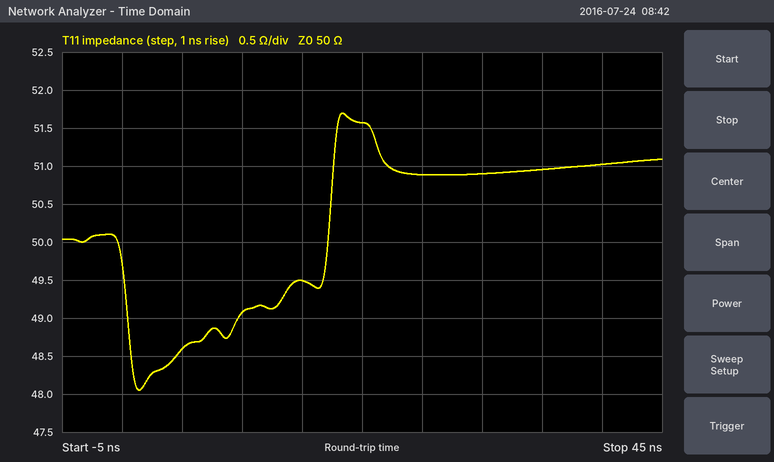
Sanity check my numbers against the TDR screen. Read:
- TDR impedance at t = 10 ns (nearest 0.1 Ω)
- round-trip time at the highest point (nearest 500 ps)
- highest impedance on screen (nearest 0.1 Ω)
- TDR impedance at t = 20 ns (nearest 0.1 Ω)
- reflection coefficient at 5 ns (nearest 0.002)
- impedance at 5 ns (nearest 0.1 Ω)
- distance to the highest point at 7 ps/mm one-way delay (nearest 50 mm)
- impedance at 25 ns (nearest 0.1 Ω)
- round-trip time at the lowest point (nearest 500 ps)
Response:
49.1 Ω
18.5 ns
51.7 Ω
51.6 Ω
-0.014
48.6 Ω
1.30 m
50.9 Ω
1.5 ns
